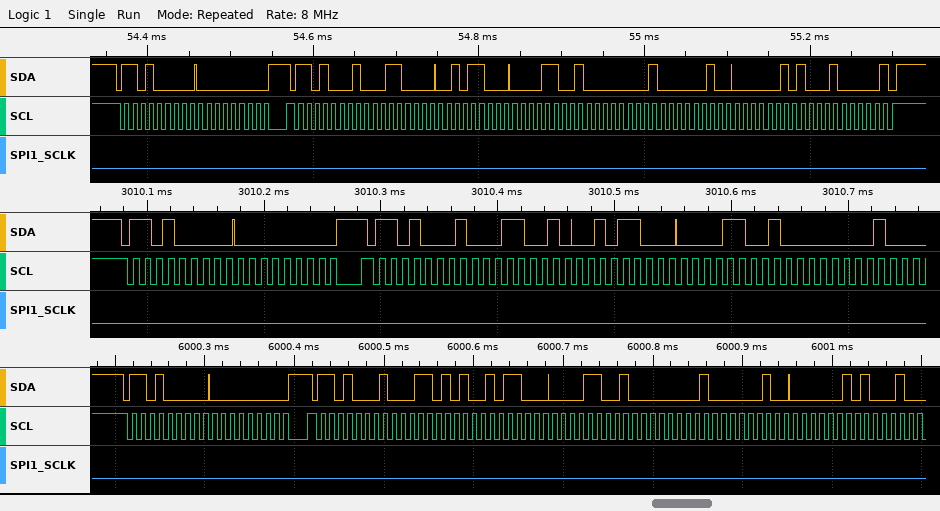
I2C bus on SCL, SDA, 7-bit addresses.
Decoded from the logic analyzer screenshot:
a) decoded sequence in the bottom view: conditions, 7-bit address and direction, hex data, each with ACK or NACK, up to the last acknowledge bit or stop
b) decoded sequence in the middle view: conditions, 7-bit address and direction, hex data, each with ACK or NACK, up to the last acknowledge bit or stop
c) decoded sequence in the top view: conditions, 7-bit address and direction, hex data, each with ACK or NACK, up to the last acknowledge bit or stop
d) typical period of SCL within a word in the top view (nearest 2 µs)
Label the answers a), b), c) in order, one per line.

a) start, address 68 write ACK, 00 ACK, repeated start, address 68 read ACK, 35 ACK, 58 ACK, 19 ACK, 01 ACK, 04 ACK, 05 ACK
b) start, address 68 write ACK, 00 ACK, repeated start, address 68 read ACK, 32 ACK, 58 ACK, 19 ACK, 01 ACK
c) start, address 68 write ACK, 00 ACK, repeated start, address 68 read ACK, 30 ACK, 58 ACK, 19 ACK, 01 ACK, 04 ACK, 05 ACK, 20 NACK, stop
d) 10 µs
